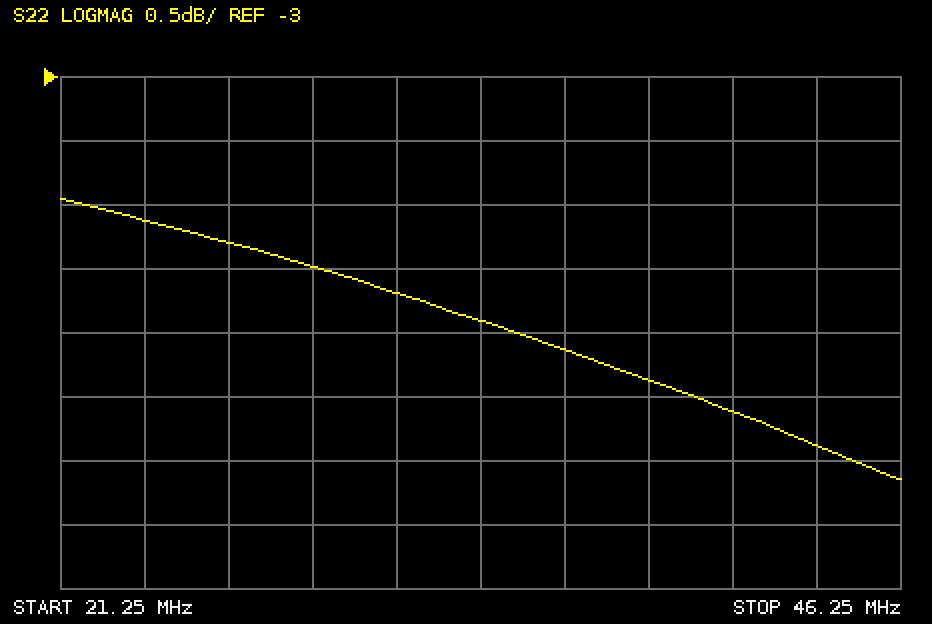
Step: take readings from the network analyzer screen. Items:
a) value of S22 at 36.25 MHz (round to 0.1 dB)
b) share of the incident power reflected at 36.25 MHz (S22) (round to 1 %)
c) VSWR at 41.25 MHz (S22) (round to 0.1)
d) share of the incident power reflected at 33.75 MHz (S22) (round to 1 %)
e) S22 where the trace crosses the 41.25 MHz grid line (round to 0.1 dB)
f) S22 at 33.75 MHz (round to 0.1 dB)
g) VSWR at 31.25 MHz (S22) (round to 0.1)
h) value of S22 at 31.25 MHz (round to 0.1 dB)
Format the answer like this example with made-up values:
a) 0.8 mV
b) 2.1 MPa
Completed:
a) -5.1 dB
b) 31 %
c) 3.2
d) 32 %
e) -5.6 dB
f) -4.9 dB
g) 3.8
h) -4.7 dB
